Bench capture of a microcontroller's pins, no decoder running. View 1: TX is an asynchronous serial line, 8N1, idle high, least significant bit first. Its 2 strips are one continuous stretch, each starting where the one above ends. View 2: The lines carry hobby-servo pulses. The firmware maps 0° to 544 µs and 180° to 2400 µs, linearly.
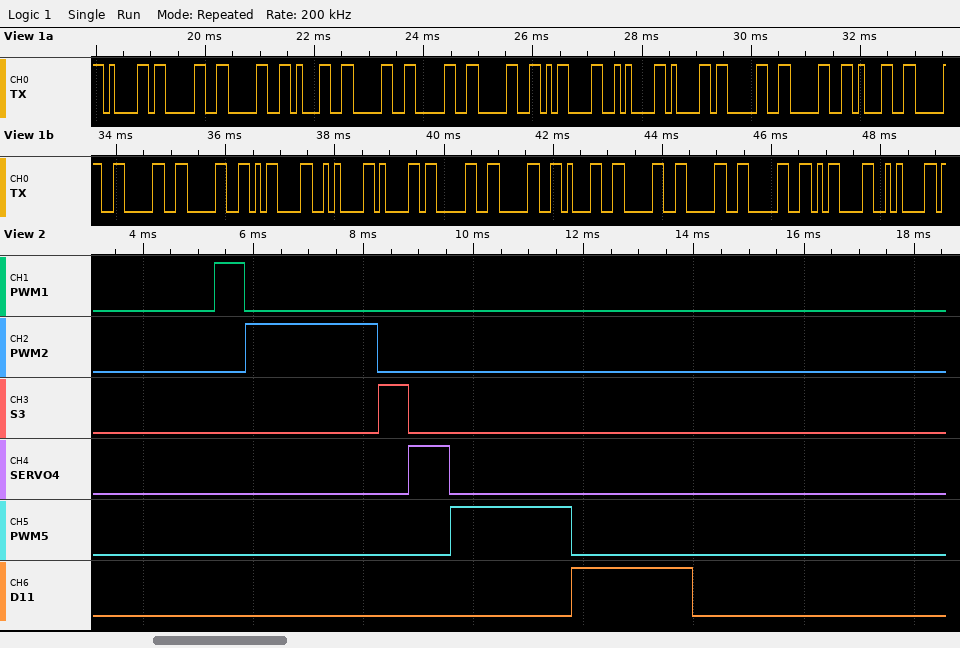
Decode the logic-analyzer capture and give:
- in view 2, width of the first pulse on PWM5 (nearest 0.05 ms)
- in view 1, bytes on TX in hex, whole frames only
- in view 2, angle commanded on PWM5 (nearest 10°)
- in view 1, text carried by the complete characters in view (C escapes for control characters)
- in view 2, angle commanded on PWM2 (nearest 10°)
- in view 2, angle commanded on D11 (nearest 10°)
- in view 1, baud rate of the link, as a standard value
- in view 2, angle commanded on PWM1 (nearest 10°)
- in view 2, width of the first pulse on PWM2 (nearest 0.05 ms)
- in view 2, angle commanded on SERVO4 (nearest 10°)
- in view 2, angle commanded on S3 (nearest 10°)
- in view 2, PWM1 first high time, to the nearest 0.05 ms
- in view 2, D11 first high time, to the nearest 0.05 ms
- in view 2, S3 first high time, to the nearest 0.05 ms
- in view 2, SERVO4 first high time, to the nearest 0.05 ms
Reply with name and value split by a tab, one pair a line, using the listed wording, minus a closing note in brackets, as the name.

in view 2, width of the first pulse on PWM5	2.20 ms
in view 1, bytes on TX in hex, whole frames only	61 30 30 31 30 30 30 0D 0A 61 30 30 31 30 30 30 0D 0A 61 30 30 31 30 30 30 0D 0A
in view 2, angle commanded on PWM5	160°
in view 1, text carried by the complete characters in view	"a001000\r\na001000\r\na001000\r\n"
in view 2, angle commanded on PWM2	180°
in view 2, angle commanded on D11	160°
in view 1, baud rate of the link, as a standard value	9600 baud
in view 2, angle commanded on PWM1	0°
in view 2, width of the first pulse on PWM2	2.40 ms
in view 2, angle commanded on SERVO4	20°
in view 2, angle commanded on S3	0°
in view 2, PWM1 first high time, to the nearest 0.05 ms	0.55 ms
in view 2, D11 first high time, to the nearest 0.05 ms	2.20 ms
in view 2, S3 first high time, to the nearest 0.05 ms	0.55 ms
in view 2, SERVO4 first high time, to the nearest 0.05 ms	0.75 ms
